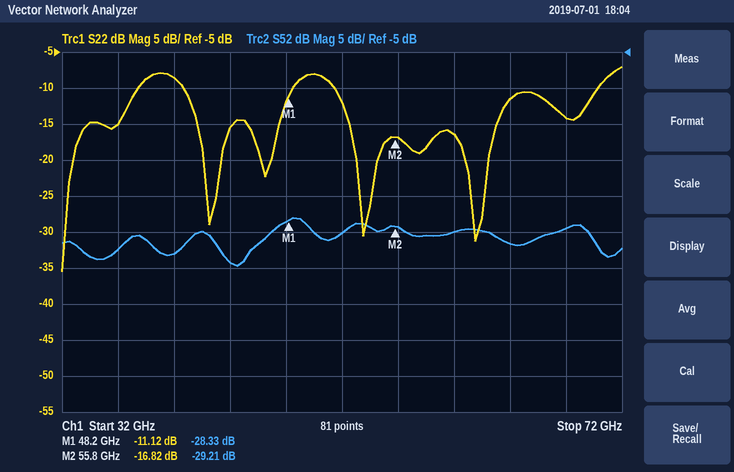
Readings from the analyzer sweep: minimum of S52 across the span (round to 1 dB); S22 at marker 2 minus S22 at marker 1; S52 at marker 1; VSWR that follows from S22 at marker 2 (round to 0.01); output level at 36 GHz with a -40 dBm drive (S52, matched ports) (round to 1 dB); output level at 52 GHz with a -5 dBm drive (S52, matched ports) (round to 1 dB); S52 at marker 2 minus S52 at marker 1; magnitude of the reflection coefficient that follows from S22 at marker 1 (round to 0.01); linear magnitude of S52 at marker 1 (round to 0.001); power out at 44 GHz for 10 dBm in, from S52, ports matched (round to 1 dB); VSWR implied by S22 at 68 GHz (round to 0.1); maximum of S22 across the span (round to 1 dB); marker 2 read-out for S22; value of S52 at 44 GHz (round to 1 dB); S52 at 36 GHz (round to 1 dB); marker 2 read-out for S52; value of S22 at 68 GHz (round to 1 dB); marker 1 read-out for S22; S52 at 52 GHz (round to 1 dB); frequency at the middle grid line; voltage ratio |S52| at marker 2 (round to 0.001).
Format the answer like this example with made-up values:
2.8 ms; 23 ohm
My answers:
-35 dB; -5.70 dB; -28.33 dB; 1.34; -72 dBm; -35 dBm; -0.88 dB; 0.28; 0.038; -24 dBm; 1.5; -7 dB; -16.82 dB; -34 dB; -32 dB; -29.21 dB; -14 dB; -11.12 dB; -30 dB; 52 GHz; 0.035
